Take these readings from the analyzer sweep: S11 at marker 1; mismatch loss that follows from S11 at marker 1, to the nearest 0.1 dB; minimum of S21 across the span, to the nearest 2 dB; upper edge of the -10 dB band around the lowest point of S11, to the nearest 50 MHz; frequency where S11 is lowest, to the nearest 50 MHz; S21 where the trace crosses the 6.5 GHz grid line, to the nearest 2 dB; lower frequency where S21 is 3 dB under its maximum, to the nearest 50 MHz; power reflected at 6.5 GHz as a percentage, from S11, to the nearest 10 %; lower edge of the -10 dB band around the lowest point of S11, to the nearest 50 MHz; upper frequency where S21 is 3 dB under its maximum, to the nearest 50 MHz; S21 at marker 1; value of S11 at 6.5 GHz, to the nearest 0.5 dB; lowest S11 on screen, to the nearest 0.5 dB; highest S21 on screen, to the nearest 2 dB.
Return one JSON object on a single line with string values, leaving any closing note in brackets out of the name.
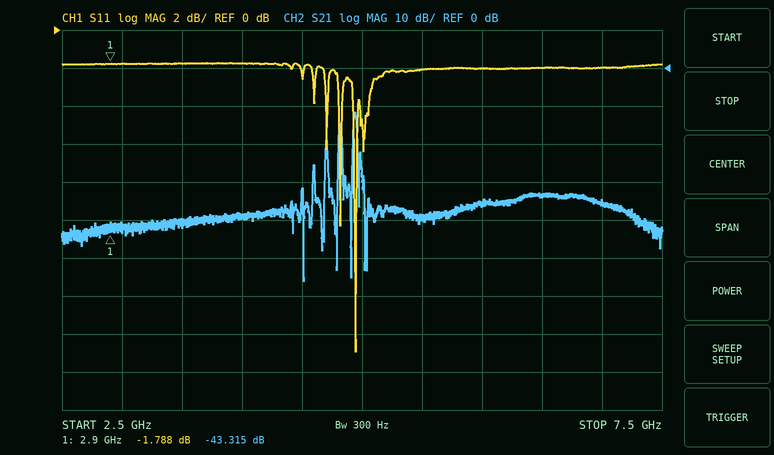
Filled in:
{"S11 at marker 1": "-1.788 dB", "mismatch loss that follows from S11 at marker 1, to the nearest 0.1 dB": "4.7 dB", "minimum of S21 across the span, to the nearest 2 dB": "-56 dB", "upper edge of the -10 dB band around the lowest point of S11, to the nearest 50 MHz": "4.95 GHz", "frequency where S11 is lowest, to the nearest 50 MHz": "4.95 GHz", "S21 where the trace crosses the 6.5 GHz grid line, to the nearest 2 dB": "-34 dB", "lower frequency where S21 is 3 dB under its maximum, to the nearest 50 MHz": "4.95 GHz", "power reflected at 6.5 GHz as a percentage, from S11, to the nearest 10 %": "60 %", "lower edge of the -10 dB band around the lowest point of S11, to the nearest 50 MHz": "4.95 GHz", "upper frequency where S21 is 3 dB under its maximum, to the nearest 50 MHz": "4.95 GHz", "S21 at marker 1": "-43.315 dB", "value of S11 at 6.5 GHz, to the nearest 0.5 dB": "-2.0 dB", "lowest S11 on screen, to the nearest 0.5 dB": "-17.0 dB", "highest S21 on screen, to the nearest 2 dB": "-12 dB"}
